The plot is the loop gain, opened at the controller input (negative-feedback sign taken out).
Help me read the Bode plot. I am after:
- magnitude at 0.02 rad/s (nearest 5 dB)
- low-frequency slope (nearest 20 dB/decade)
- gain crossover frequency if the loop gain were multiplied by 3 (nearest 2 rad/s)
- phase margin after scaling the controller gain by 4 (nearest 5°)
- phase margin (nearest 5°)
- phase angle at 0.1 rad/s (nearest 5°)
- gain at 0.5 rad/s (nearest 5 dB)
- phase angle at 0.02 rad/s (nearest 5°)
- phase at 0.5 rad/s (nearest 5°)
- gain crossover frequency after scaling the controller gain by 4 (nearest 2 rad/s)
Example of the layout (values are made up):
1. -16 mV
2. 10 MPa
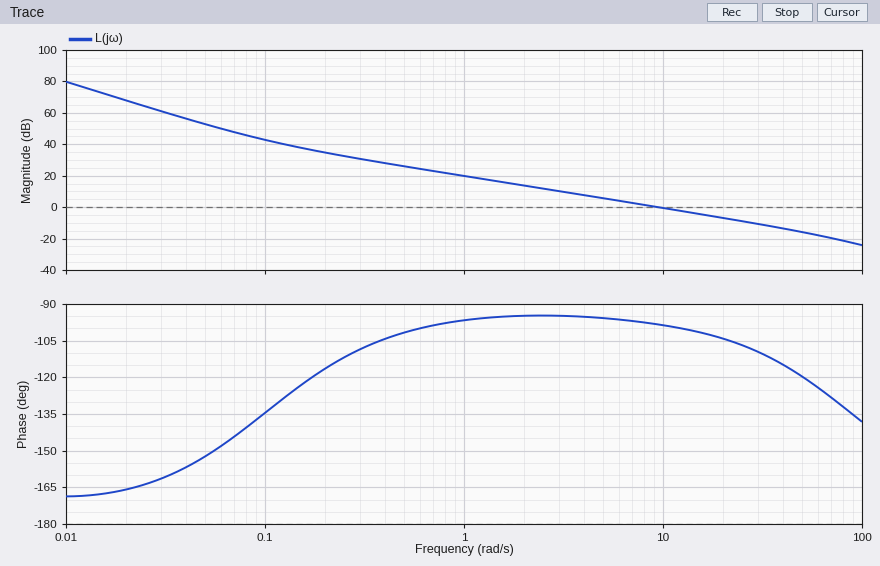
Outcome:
1. 70 dB
2. -40 dB/decade
3. 26 rad/s
4. 70°
5. 80°
6. -135°
7. 25 dB
8. -165°
9. -100°
10. 34 rad/s
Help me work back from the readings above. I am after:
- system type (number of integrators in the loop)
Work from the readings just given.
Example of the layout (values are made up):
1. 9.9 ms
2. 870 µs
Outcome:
1. 2
